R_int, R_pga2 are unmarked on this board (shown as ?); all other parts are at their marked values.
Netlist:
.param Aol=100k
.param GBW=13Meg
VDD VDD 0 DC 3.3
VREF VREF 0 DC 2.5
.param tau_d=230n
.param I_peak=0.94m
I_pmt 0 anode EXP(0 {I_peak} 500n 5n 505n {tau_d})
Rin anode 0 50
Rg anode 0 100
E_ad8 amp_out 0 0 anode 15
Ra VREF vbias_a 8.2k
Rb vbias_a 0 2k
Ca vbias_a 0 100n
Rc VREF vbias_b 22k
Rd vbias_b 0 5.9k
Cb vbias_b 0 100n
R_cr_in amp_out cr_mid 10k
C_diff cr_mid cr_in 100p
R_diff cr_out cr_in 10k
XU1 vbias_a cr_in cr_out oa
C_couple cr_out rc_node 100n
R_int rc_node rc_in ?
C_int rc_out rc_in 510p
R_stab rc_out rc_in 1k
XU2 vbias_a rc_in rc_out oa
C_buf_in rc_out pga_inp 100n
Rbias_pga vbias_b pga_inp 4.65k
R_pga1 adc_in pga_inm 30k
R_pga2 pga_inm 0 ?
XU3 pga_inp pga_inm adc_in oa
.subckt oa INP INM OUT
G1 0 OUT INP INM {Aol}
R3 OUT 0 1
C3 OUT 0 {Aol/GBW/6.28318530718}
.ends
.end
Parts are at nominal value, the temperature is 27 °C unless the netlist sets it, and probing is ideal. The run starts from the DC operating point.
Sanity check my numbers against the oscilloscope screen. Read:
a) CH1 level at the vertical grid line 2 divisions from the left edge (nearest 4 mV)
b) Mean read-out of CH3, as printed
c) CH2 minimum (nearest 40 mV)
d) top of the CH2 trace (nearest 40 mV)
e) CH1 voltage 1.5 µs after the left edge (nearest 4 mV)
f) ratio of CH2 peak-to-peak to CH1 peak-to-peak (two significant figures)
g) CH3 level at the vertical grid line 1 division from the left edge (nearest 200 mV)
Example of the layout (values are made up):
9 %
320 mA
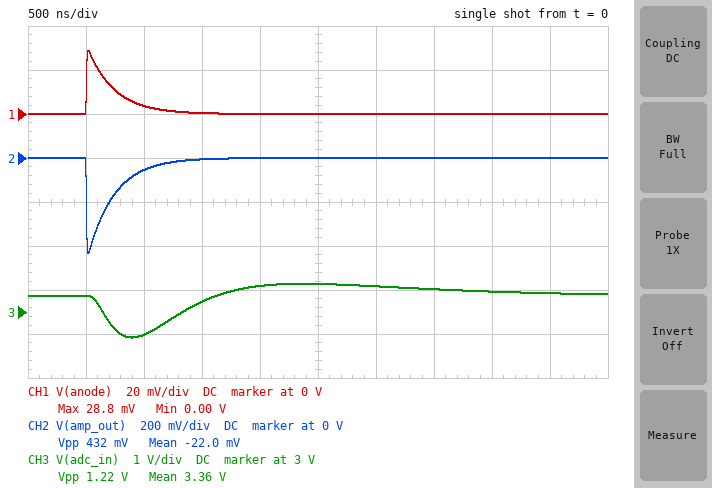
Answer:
4 mV
3.36 V
-440 mV
0 V
0 V
15
3.4 V
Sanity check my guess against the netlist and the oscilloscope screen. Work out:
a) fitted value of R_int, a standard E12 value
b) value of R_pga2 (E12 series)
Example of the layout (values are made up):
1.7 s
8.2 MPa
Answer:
560 Ω
5.6 kΩ
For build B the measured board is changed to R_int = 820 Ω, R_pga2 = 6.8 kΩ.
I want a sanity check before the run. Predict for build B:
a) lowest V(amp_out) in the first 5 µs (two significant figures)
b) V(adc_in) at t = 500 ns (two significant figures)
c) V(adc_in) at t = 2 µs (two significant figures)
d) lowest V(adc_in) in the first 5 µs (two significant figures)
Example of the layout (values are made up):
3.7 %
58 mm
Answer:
-430 mV
2.9 V
3.0 V
2.3 V
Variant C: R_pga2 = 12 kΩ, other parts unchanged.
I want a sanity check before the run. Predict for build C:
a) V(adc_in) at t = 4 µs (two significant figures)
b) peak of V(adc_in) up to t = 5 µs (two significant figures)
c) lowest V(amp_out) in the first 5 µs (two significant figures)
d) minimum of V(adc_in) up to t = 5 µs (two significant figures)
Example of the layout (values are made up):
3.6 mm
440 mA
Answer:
1.9 V
2.0 V
-430 mV
1.3 V
